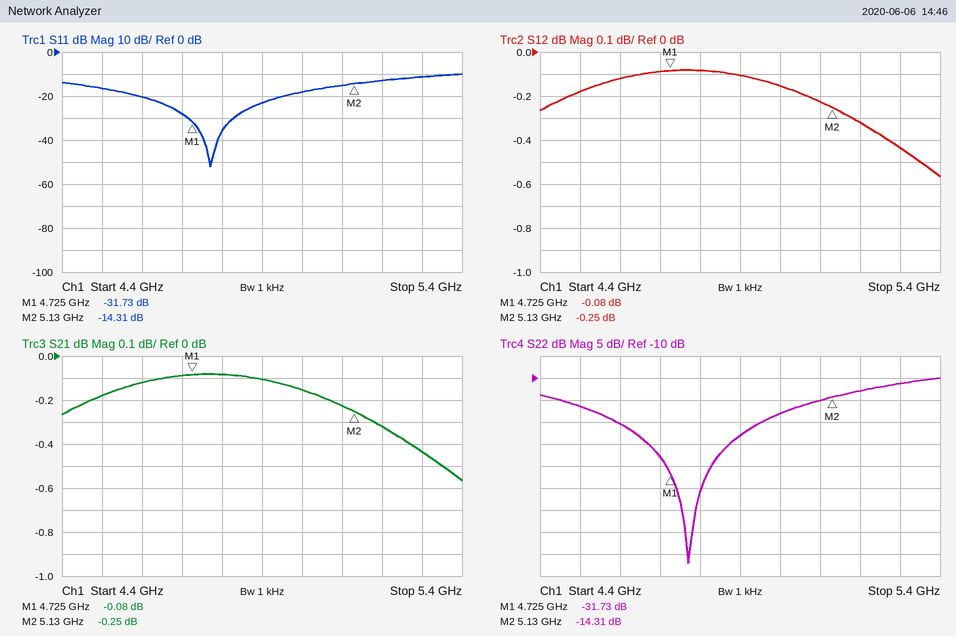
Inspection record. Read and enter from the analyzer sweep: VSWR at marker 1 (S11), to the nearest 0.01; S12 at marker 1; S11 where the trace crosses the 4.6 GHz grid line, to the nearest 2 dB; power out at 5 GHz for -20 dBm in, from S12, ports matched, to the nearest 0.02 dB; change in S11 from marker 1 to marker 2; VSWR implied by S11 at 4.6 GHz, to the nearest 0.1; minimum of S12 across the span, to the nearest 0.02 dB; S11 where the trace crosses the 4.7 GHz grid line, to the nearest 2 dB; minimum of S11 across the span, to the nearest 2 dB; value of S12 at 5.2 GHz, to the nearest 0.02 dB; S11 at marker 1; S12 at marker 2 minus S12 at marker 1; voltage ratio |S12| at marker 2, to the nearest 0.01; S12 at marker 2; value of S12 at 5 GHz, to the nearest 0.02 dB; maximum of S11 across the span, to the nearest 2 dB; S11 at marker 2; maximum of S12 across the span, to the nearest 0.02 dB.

1.05
-0.08 dB
-20 dB
-20.16 dBm
17.42 dB
1.2
-0.56 dB
-28 dB
-52 dB
-0.32 dB
-31.73 dB
-0.17 dB
0.97
-0.25 dB
-0.16 dB
-10 dB
-14.31 dB
-0.08 dB
